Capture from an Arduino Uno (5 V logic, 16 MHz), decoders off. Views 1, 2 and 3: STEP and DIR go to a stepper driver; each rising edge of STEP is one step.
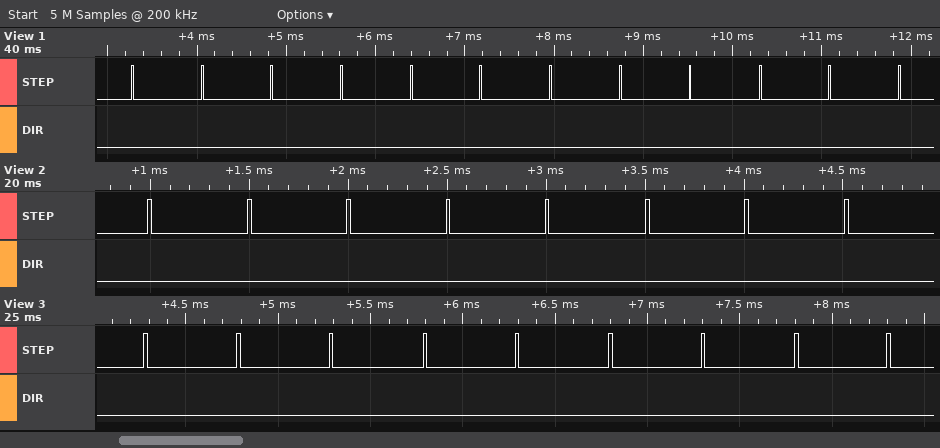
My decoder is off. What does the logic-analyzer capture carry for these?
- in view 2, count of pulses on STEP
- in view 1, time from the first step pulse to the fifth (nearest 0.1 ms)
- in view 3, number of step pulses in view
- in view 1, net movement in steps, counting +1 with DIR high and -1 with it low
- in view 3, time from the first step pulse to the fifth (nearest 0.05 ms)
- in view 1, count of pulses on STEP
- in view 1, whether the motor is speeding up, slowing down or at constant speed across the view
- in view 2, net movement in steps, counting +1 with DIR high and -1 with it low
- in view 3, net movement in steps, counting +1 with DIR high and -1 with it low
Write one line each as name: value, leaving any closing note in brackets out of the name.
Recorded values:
in view 2, count of pulses on STEP: 8
in view 1, time from the first step pulse to the fifth: 3.1 ms
in view 3, number of step pulses in view: 9
in view 1, net movement in steps, counting +1 with DIR high and -1 with it low: -12
in view 3, time from the first step pulse to the fifth: 2.00 ms
in view 1, count of pulses on STEP: 12
in view 1, whether the motor is speeding up, slowing down or at constant speed across the view: constant speed
in view 2, net movement in steps, counting +1 with DIR high and -1 with it low: -8
in view 3, net movement in steps, counting +1 with DIR high and -1 with it low: -9
